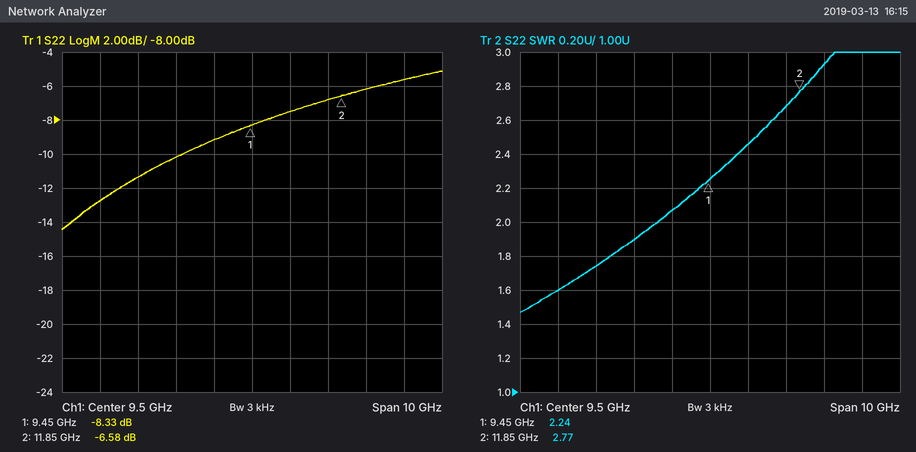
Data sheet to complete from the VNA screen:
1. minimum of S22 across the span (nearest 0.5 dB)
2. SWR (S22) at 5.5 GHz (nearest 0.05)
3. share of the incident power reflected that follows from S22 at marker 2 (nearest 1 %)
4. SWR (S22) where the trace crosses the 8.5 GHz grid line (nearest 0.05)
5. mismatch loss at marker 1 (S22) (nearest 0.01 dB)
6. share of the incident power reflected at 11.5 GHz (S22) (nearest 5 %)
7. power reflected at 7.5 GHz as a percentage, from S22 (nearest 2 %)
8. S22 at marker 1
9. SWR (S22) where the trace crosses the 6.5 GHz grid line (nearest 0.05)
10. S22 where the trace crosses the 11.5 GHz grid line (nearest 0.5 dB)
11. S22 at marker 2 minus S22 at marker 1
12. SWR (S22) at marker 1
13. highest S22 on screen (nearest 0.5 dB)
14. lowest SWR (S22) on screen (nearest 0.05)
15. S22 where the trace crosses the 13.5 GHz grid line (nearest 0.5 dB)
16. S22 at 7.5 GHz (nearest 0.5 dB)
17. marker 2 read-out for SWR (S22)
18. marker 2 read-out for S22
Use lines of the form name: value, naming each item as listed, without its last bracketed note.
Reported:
minimum of S22 across the span: -14.5 dB
SWR (S22) at 5.5 GHz: 1.60
share of the incident power reflected that follows from S22 at marker 2: 22 %
SWR (S22) where the trace crosses the 8.5 GHz grid line: 2.05
mismatch loss at marker 1 (S22): 0.69 dB
share of the incident power reflected at 11.5 GHz (S22): 20 %
power reflected at 7.5 GHz as a percentage, from S22: 10 %
S22 at marker 1: -8.33 dB
SWR (S22) where the trace crosses the 6.5 GHz grid line: 1.75
S22 where the trace crosses the 11.5 GHz grid line: -7.0 dB
S22 at marker 2 minus S22 at marker 1: 1.75 dB
SWR (S22) at marker 1: 2.24
highest S22 on screen: -5.0 dB
lowest SWR (S22) on screen: 1.45
S22 where the trace crosses the 13.5 GHz grid line: -5.5 dB
S22 at 7.5 GHz: -10.0 dB
marker 2 read-out for SWR: 2.77
marker 2 read-out for S22: -6.58 dB
